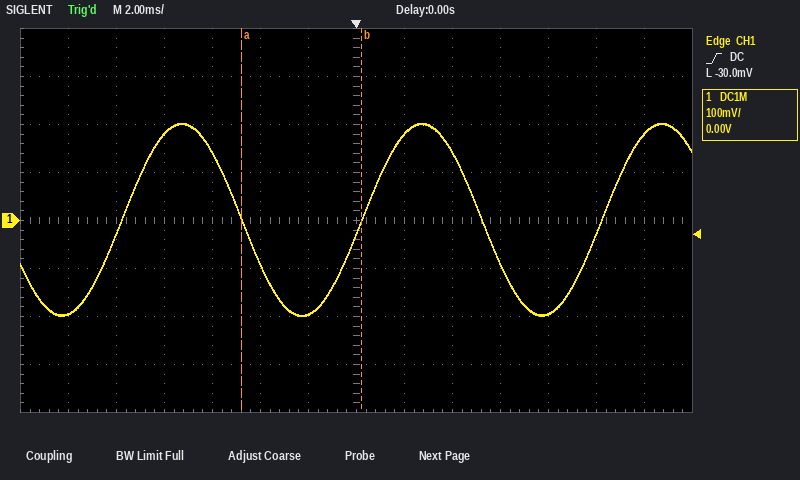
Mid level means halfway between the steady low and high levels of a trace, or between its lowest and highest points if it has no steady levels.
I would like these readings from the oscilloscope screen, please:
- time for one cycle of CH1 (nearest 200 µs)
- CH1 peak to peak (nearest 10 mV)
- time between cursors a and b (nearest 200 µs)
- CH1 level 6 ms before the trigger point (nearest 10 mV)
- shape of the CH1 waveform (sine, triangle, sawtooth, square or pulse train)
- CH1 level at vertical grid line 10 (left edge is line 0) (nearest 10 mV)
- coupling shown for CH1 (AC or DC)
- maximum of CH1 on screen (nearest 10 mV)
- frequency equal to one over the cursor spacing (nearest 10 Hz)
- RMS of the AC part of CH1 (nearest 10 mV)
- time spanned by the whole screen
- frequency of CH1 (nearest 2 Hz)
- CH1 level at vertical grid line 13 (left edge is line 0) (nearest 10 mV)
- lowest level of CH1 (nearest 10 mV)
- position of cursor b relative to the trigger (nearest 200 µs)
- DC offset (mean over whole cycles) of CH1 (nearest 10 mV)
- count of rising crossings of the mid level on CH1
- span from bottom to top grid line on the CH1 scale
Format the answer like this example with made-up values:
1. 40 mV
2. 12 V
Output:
1. 10.0 ms
2. 400 mV
3. 5.0 ms
4. 140 mV
5. sine
6. -90 mV
7. DC
8. 200 mV
9. 200 Hz
10. 140 mV
11. 28 ms
12. 100 Hz
13. 180 mV
14. -200 mV
15. +200 µs
16. 0 mV
17. 3
18. 800 mV
